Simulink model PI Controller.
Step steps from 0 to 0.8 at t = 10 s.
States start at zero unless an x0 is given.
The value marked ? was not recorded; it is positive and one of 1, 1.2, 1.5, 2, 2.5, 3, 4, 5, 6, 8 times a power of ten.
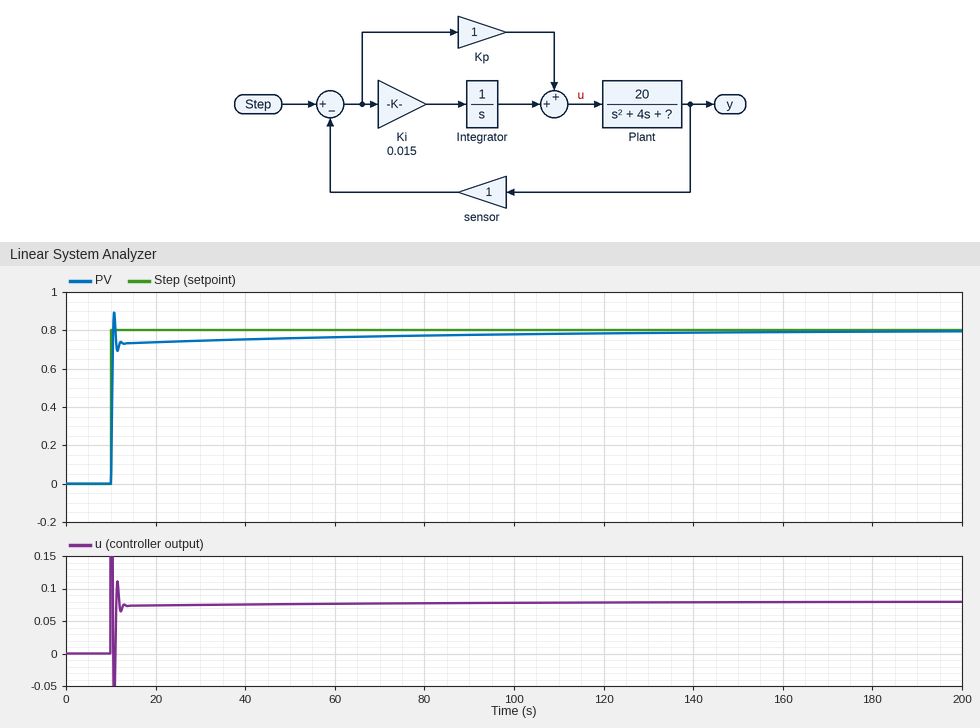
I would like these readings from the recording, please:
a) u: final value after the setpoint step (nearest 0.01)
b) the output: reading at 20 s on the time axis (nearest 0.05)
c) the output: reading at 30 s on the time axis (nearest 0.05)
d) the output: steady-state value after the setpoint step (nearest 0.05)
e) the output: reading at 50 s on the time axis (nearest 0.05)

0.08
0.75
0.75
0.80
0.75
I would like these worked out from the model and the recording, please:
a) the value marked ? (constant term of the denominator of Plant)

2
